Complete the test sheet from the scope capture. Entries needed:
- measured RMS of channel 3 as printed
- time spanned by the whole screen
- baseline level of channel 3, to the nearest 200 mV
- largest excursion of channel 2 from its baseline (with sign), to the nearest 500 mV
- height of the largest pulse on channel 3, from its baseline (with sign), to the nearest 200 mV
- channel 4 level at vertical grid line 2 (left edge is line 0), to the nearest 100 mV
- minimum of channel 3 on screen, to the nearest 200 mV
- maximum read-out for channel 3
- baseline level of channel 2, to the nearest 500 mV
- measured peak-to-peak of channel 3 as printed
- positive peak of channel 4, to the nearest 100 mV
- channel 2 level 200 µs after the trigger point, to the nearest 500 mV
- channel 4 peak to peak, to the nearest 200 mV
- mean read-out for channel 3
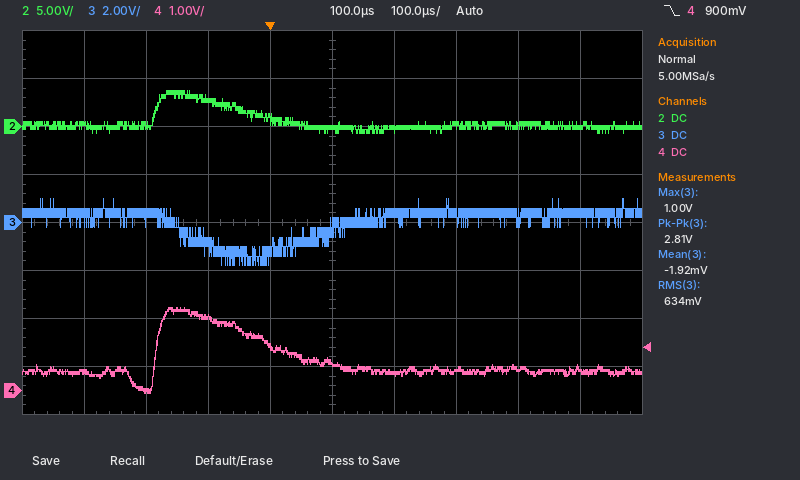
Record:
634 mV
1 ms
400 mV
+4.0 V
-2.2 V
0.0 V
-1.8 V
1.00 V
0.0 V
2.81 V
1.7 V
-500 mV
1.8 V
-1.92 mV
